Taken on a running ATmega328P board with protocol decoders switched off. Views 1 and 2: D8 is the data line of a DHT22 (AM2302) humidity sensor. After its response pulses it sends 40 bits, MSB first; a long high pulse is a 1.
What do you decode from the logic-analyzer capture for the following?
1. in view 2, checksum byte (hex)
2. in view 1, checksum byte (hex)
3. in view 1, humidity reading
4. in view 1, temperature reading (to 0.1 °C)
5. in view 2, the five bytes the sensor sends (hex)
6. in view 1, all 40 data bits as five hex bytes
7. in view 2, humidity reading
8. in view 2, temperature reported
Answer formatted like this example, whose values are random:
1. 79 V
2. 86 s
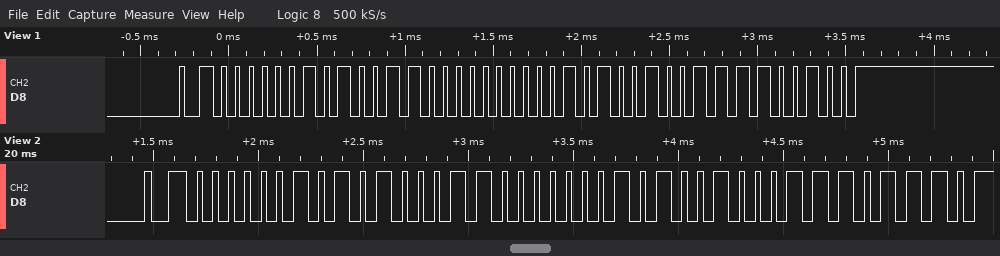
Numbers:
1. 0xEE
2. 0xE4
3. 66.4 %
4. 32.9 °C
5. 02 A3 01 48 EE
6. 02 98 01 49 E4
7. 67.5 %
8. 32.8 °C
